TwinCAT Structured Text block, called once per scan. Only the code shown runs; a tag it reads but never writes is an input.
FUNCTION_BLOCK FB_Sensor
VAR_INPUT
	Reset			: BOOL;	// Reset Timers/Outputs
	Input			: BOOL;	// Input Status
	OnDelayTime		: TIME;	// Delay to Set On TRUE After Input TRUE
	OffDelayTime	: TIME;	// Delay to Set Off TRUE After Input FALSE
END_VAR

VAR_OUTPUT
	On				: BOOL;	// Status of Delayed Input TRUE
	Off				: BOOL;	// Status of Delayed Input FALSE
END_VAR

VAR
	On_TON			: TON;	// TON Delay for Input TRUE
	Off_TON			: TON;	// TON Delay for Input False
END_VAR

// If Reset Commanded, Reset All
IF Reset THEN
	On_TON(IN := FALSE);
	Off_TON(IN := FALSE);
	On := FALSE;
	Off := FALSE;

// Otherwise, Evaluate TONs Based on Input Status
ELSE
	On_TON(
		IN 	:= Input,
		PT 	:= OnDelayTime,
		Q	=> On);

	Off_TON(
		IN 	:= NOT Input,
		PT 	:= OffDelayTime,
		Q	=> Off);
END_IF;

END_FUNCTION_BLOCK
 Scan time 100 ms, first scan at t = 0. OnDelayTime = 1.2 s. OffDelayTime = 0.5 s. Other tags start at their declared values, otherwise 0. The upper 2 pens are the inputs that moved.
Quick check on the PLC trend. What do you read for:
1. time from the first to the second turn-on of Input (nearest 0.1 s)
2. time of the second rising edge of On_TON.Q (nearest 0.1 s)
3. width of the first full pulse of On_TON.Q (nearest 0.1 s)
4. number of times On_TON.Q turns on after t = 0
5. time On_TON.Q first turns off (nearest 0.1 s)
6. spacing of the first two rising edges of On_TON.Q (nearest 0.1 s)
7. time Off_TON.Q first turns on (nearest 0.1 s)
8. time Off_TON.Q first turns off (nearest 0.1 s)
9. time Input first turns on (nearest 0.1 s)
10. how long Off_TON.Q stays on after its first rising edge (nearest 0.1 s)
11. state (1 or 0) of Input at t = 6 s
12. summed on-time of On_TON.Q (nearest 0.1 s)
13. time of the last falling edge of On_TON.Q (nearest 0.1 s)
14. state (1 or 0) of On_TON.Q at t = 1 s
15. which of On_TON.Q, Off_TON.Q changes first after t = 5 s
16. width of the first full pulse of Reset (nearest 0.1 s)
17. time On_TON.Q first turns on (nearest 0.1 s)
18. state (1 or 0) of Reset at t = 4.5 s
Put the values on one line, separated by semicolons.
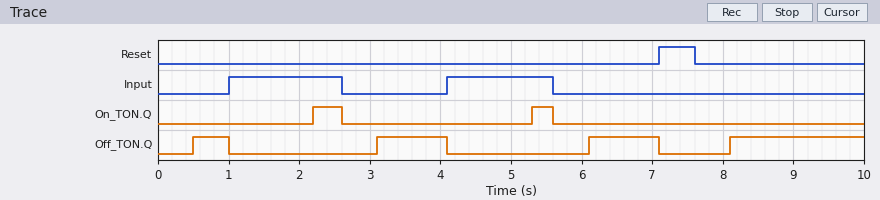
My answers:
3.1 s; 5.3 s; 0.4 s; 2; 2.6 s; 3.1 s; 0.5 s; 1.0 s; 1.0 s; 0.5 s; 0; 0.7 s; 5.6 s; 0; On_TON.Q; 0.5 s; 2.2 s; 0
